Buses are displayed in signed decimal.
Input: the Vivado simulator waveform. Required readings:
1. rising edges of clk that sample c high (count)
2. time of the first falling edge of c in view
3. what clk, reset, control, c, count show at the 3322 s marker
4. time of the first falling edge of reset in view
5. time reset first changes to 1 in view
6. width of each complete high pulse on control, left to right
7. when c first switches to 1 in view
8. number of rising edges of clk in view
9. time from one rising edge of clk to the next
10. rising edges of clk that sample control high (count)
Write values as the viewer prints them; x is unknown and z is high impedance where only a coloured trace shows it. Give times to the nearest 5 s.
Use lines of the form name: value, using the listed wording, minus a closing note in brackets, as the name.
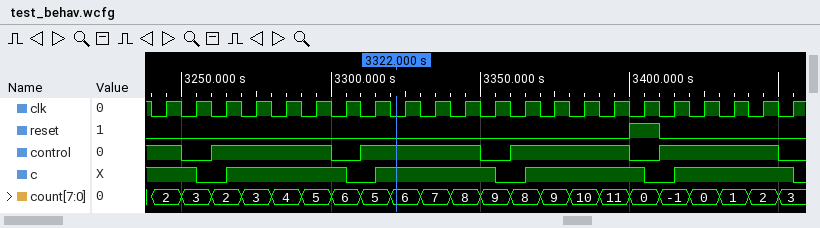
rising edges of clk that sample c high: 18
time of the first falling edge of c in view: 3255 s
what clk, reset, control, c, count show at the 3322 s marker: clk=0, reset=0, control=1, c=1, count=6
time of the first falling edge of reset in view: 3410 s
time reset first changes to 1 in view: 3400 s
width of each complete high pulse on control, left to right: 40 s, 40 s, 40 s, 40 s
when c first switches to 1 in view: 3265 s
number of rising edges of clk in view: 22
time from one rising edge of clk to the next: 10 s
rising edges of clk that sample control high: 17
